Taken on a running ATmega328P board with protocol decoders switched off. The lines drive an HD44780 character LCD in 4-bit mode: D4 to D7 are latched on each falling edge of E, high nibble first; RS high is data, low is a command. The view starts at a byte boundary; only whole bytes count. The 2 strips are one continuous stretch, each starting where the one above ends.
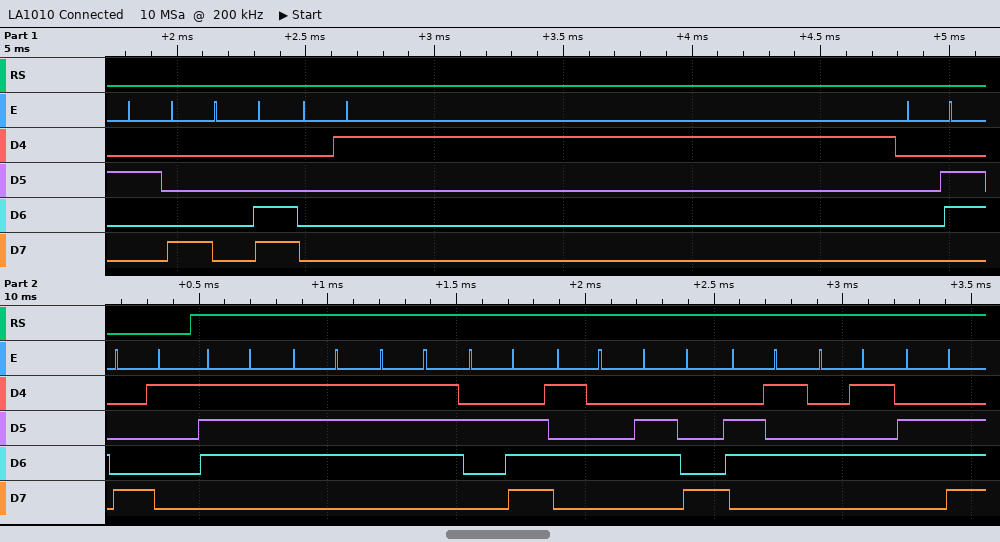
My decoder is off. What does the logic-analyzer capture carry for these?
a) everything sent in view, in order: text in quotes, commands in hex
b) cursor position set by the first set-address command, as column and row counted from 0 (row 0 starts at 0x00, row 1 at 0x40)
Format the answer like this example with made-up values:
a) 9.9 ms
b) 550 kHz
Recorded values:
a) 0x28 0x0C 0x01 0x06 0x81 "www.TheEn"
b) column 1, row 0
